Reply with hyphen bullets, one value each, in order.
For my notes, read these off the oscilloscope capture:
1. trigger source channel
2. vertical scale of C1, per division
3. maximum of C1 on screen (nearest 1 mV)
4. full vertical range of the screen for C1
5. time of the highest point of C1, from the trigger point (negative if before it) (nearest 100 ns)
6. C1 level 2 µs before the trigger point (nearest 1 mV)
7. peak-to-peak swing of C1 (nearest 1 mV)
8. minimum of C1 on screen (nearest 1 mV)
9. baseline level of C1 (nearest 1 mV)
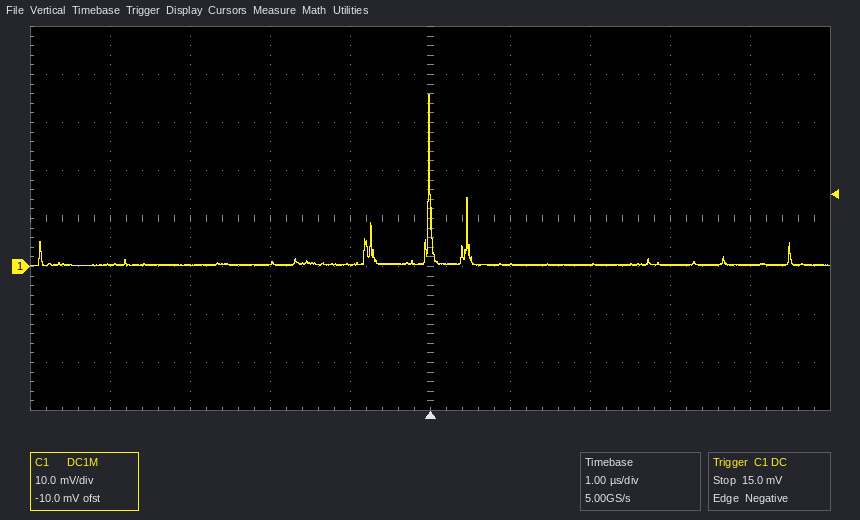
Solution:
- C1
- 10 mV
- 36 mV
- 80 mV
- 0.0 µs
- 1 mV
- 36 mV
- 0 mV
- 0 mV
